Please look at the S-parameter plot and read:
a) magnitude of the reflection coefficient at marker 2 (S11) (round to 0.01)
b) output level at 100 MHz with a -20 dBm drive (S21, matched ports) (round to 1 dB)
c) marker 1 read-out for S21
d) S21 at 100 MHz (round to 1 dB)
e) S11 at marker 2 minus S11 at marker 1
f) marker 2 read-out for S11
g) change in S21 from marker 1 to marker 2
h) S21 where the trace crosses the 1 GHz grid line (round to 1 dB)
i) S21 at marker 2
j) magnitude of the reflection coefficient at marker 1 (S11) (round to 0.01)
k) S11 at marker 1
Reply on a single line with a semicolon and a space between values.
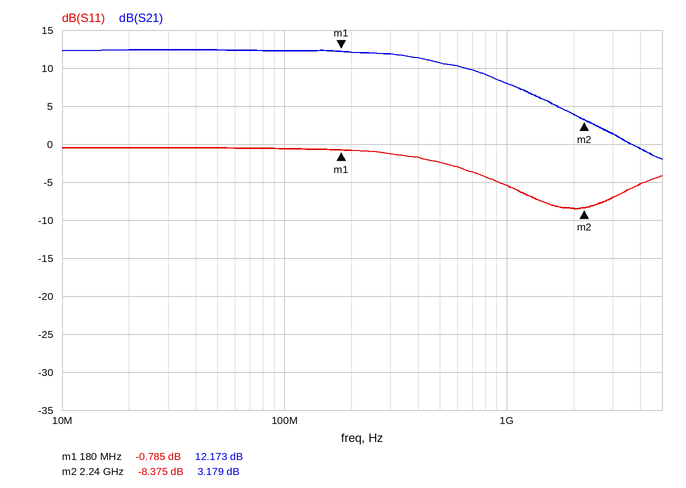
0.38; -8 dBm; 12.173 dB; 12 dB; -7.590 dB; -8.375 dB; -8.994 dB; 8 dB; 3.179 dB; 0.91; -0.785 dB
